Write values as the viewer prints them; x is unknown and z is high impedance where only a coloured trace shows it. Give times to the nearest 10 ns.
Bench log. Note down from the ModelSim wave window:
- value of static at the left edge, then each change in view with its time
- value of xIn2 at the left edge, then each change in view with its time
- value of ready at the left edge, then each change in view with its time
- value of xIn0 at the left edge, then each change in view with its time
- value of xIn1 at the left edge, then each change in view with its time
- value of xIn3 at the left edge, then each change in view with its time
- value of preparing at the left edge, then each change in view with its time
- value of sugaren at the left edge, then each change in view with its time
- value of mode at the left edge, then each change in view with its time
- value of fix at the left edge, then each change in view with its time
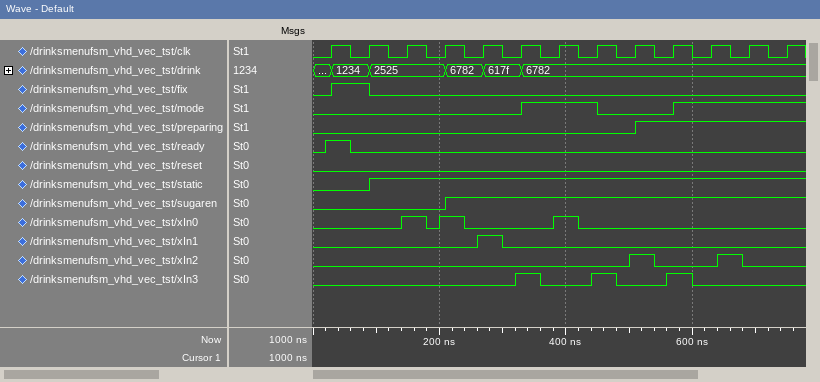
0, 1 at 90 ns
0, 1 at 500 ns, 0 at 540 ns, 1 at 640 ns, 0 at 680 ns
0, 1 at 20 ns, 0 at 60 ns
0, 1 at 140 ns, 0 at 180 ns, 1 at 200 ns, 0 at 240 ns, 1 at 380 ns, 0 at 420 ns
0, 1 at 260 ns, 0 at 300 ns
0, 1 at 320 ns, 0 at 360 ns, 1 at 440 ns, 0 at 480 ns, 1 at 560 ns, 0 at 600 ns
0, 1 at 510 ns
0, 1 at 210 ns
0, 1 at 330 ns, 0 at 450 ns, 1 at 570 ns
0, 1 at 30 ns, 0 at 90 ns
